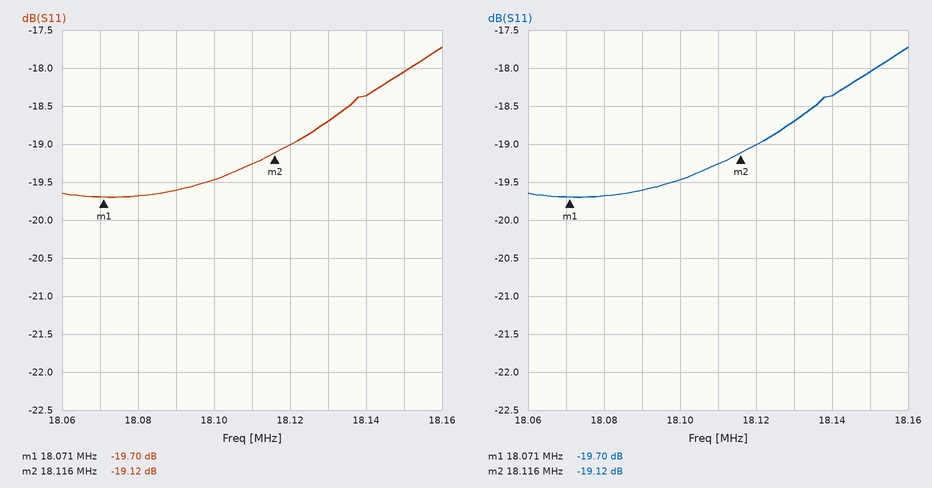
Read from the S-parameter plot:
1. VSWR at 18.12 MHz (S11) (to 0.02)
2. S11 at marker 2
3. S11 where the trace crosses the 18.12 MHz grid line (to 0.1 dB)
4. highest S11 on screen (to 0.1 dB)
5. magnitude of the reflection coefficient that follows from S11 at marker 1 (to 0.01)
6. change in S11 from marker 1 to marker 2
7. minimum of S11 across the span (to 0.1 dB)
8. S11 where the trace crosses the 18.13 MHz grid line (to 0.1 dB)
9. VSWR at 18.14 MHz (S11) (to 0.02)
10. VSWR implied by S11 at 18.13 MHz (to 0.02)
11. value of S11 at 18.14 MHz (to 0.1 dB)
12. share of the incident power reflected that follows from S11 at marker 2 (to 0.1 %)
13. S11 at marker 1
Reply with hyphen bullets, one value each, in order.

- 1.26
- -19.12 dB
- -19.0 dB
- -17.7 dB
- 0.10
- 0.58 dB
- -19.7 dB
- -18.7 dB
- 1.28
- 1.26
- -18.4 dB
- 1.2 %
- -19.70 dB
